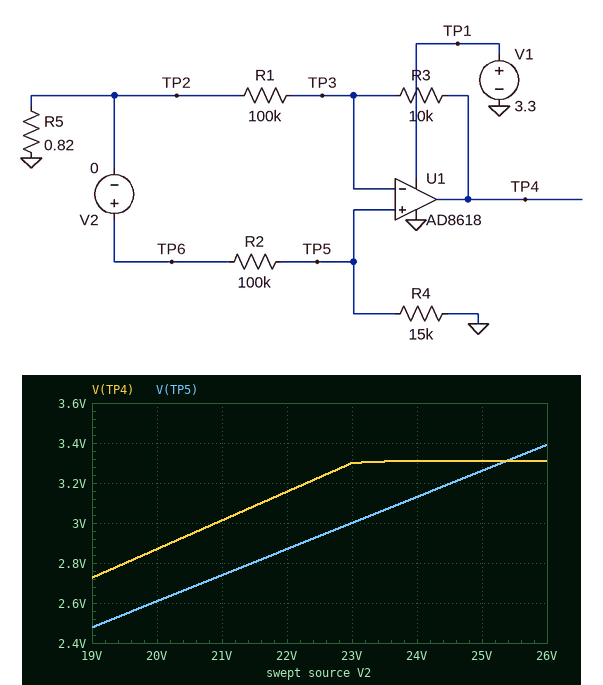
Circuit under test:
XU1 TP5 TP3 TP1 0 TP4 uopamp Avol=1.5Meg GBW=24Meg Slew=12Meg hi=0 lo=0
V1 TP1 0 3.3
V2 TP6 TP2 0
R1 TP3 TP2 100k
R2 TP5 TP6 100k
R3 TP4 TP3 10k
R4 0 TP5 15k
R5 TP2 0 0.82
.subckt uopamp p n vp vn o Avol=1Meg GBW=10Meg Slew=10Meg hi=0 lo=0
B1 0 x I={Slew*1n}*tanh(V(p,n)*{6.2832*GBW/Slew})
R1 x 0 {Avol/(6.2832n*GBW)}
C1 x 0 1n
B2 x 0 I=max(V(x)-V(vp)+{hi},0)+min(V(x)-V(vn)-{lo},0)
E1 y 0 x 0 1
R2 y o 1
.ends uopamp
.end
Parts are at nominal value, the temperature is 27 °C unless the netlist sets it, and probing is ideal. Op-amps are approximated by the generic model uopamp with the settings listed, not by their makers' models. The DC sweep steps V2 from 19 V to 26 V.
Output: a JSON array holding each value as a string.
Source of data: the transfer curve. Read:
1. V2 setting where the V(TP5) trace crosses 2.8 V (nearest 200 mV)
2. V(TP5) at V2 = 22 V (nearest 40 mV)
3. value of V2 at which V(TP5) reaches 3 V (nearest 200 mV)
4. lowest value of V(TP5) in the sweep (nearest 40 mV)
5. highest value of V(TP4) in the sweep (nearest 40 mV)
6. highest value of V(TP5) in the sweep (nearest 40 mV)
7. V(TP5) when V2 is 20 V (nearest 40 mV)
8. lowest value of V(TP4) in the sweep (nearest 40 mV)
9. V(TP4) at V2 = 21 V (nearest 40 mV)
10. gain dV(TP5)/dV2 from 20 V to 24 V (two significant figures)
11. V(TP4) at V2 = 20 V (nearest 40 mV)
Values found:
["21.4 V", "2.88 V", "23.0 V", "2.48 V", "3.32 V", "3.40 V", "2.60 V", "2.72 V", "3.00 V", "0.13 V/V", "2.88 V"]
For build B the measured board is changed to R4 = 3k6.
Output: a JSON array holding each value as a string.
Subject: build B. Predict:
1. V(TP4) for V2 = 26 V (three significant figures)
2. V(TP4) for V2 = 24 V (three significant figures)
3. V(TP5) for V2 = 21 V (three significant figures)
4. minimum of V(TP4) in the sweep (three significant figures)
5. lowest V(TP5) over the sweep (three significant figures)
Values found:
["994 mV", "917 mV", "730 mV", "726 mV", "660 mV"]
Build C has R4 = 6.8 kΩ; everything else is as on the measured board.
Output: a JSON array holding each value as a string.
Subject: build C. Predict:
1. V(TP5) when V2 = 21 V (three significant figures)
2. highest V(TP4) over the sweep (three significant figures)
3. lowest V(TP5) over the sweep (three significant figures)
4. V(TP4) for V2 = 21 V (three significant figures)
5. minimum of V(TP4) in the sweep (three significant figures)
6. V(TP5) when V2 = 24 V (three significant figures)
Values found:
["1.34 V", "1.82 V", "1.21 V", "1.47 V", "1.33 V", "1.53 V"]
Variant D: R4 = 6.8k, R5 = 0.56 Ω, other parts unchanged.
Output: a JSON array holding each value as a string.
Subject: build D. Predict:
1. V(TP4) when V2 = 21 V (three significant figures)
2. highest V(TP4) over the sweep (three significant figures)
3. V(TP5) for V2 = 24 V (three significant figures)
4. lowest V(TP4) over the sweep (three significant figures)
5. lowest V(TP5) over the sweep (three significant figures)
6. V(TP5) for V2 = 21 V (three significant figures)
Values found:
["1.47 V", "1.82 V", "1.53 V", "1.33 V", "1.21 V", "1.34 V"]
